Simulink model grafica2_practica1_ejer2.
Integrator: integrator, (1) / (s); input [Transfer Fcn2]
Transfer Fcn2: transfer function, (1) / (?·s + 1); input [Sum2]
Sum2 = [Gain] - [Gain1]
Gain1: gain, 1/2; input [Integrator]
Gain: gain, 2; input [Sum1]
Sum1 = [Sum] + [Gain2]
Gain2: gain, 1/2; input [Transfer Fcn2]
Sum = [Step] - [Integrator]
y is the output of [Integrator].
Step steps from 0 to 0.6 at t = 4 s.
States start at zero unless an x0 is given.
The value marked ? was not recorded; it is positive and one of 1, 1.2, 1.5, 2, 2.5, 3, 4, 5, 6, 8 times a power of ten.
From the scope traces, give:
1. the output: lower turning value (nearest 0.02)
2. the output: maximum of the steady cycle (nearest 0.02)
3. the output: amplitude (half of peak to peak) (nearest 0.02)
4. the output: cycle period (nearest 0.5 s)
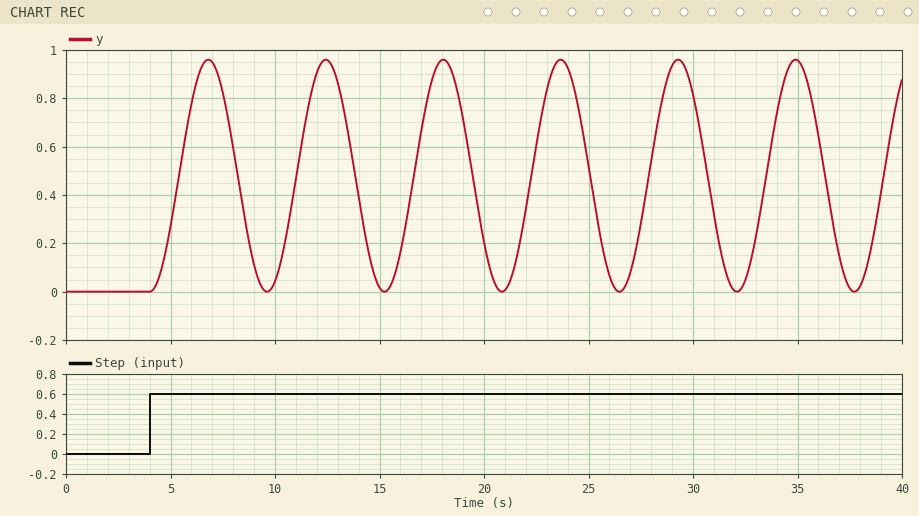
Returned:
0.00
0.96
0.48
5.5 s
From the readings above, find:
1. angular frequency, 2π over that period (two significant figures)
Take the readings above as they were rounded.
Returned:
1.1 rad/s
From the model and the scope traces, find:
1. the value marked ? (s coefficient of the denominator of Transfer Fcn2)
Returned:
2
